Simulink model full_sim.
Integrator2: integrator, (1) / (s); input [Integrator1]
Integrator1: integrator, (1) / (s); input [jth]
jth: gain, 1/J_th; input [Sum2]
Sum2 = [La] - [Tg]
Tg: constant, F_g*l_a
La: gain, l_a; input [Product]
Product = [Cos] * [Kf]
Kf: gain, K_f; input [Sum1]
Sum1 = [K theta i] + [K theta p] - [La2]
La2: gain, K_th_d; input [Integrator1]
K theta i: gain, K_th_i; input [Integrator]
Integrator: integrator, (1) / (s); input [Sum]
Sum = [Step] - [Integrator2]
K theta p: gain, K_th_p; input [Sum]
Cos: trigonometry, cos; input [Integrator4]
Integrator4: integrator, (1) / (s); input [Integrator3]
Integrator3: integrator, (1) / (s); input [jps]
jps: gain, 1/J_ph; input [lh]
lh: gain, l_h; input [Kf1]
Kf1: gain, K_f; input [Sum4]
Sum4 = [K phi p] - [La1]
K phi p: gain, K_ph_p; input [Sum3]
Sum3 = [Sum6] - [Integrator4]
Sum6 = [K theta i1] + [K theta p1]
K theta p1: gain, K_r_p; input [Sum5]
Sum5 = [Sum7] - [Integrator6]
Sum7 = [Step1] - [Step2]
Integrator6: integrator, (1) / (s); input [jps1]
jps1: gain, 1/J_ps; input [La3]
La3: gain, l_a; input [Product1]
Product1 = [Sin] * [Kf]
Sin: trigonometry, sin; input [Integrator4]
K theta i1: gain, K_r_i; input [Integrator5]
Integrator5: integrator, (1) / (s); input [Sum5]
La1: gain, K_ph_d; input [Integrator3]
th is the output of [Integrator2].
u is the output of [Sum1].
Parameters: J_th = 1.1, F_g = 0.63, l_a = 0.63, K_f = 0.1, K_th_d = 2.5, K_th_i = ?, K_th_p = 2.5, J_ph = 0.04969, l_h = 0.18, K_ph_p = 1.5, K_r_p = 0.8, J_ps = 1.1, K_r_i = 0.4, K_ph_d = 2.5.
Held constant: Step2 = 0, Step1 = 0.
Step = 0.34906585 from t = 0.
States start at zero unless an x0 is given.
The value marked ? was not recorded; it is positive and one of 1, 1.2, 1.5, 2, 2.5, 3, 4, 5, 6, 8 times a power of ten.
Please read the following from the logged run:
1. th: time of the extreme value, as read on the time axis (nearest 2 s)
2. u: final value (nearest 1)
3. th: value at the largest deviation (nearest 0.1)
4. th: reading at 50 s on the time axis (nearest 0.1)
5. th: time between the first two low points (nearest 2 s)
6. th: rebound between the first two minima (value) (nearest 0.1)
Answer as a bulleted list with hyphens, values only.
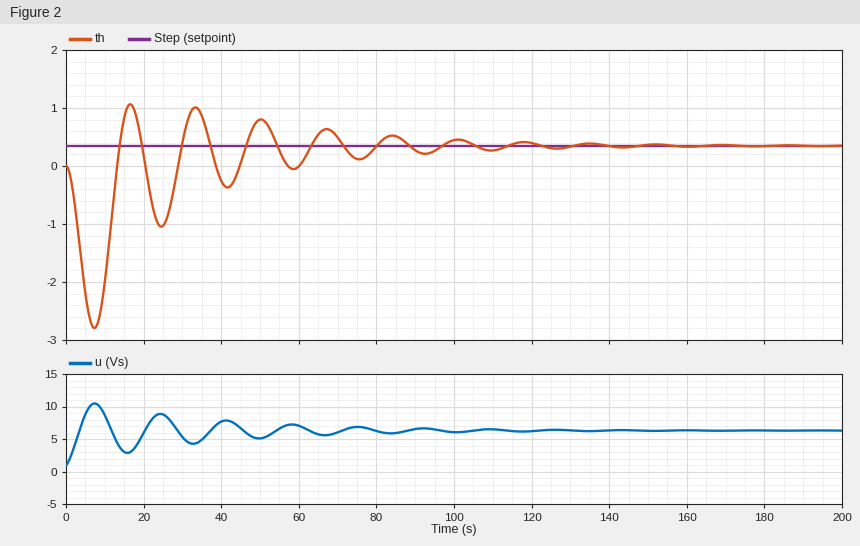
- 8 s
- 6
- -2.8
- 0.8
- 18 s
- 1.1
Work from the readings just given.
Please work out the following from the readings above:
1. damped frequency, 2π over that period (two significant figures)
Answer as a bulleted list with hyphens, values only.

- 0.35 rad/s
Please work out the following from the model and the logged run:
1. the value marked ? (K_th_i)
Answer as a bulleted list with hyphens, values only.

- 0.2
